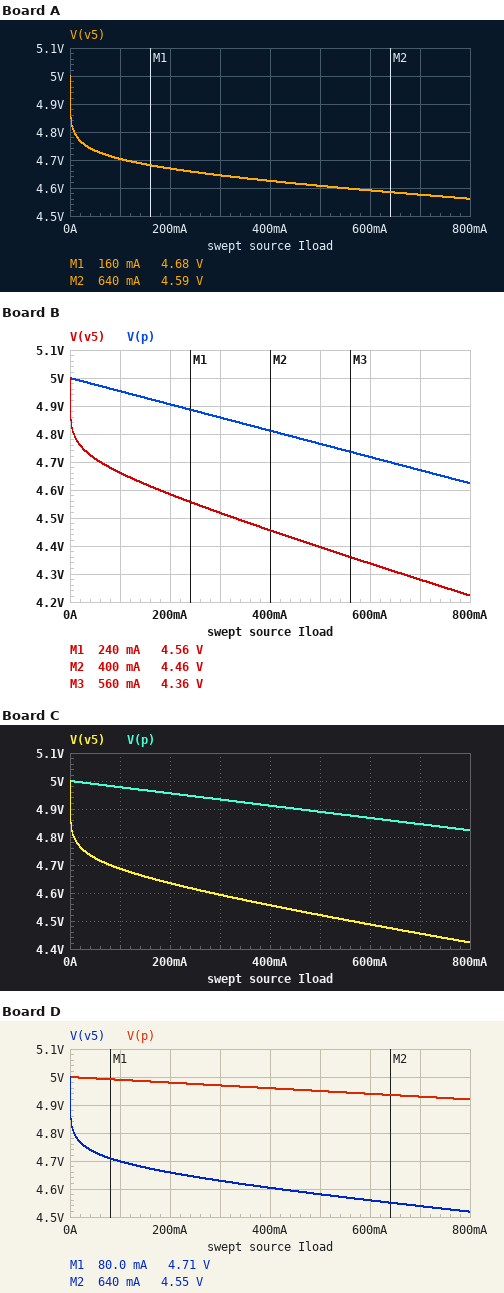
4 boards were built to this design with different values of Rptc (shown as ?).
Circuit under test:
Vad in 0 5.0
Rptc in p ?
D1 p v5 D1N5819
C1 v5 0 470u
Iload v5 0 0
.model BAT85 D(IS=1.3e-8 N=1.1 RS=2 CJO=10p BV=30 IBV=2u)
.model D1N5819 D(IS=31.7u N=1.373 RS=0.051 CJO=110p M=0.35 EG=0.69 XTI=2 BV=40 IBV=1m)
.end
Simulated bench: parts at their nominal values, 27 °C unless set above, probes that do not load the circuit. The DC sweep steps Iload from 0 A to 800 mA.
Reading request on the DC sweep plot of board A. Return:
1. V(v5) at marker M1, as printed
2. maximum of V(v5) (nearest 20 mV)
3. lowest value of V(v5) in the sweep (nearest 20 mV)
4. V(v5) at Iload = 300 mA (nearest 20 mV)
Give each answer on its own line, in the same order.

4.68 V
5.00 V
4.56 V
4.64 V
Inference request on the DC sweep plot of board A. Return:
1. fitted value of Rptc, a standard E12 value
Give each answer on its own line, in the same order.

0.047 Ω
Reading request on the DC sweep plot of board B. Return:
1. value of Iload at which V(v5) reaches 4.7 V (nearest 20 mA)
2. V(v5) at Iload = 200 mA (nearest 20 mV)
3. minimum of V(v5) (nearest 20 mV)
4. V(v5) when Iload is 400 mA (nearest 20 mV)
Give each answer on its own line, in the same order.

60 mA
4.58 V
4.22 V
4.46 V
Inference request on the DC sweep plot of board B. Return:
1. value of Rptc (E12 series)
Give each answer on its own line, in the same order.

0.47 Ω
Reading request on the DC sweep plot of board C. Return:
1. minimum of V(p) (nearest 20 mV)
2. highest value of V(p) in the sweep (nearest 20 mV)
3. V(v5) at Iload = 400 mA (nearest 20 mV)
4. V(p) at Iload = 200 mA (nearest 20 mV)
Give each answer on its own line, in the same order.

4.82 V
5.00 V
4.56 V
4.96 V
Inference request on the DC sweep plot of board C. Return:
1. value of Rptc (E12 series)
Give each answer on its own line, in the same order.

0.22 Ω
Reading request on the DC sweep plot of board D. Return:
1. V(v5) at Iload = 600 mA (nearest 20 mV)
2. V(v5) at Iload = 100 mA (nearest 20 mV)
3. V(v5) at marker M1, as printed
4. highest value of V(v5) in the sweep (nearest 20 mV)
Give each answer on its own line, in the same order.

4.56 V
4.70 V
4.71 V
5.00 V
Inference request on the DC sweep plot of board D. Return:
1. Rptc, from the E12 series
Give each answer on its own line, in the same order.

0.1 Ω
